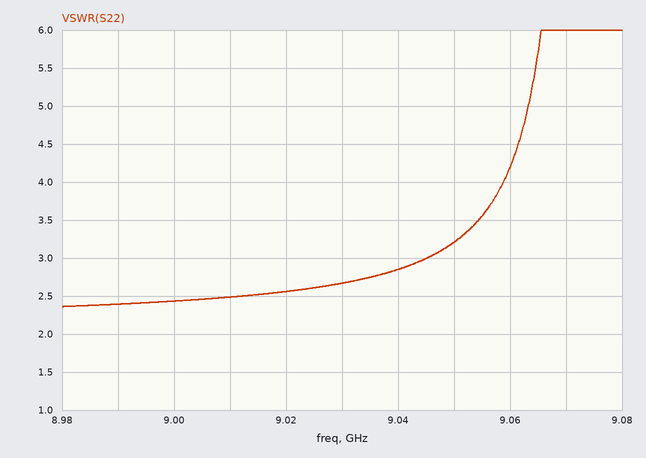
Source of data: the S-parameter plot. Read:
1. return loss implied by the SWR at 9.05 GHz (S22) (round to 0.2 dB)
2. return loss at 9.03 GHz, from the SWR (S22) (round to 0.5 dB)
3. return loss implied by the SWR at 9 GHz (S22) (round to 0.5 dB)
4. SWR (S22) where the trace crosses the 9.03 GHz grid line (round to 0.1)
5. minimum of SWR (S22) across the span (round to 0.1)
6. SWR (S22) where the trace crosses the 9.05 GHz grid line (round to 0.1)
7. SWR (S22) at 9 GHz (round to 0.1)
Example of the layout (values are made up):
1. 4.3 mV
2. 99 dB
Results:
1. 5.6 dB
2. 7.0 dB
3. 7.5 dB
4. 2.7
5. 2.4
6. 3.2
7. 2.4
